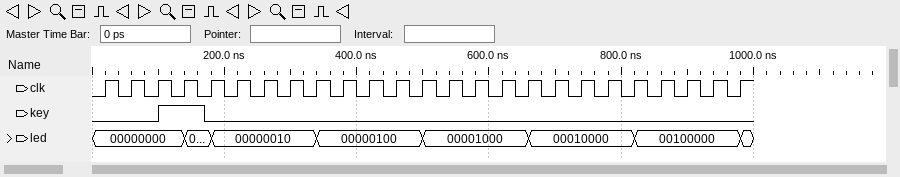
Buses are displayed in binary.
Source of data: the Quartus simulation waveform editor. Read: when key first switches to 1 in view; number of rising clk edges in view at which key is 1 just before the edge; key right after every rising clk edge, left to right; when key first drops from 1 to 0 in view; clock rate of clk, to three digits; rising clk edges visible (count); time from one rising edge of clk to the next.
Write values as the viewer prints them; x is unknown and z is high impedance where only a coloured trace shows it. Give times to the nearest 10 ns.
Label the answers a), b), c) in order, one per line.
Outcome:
a) 100 ns
b) 1
c) 0 0 1 1 0 0 0 0 0 0 0 0 0 0 0 0 0 0 0 0 0 0 0 0 0
d) 170 ns
e) 25.0 MHz
f) 25
g) 40 ns
